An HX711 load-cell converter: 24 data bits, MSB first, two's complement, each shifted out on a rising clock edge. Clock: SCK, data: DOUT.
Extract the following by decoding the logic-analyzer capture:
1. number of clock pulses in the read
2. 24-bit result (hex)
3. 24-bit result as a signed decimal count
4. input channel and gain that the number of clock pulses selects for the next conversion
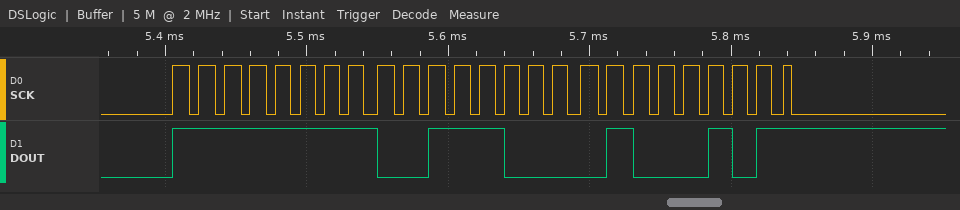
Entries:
25
0xFF3845
-51131
channel A, gain 128
